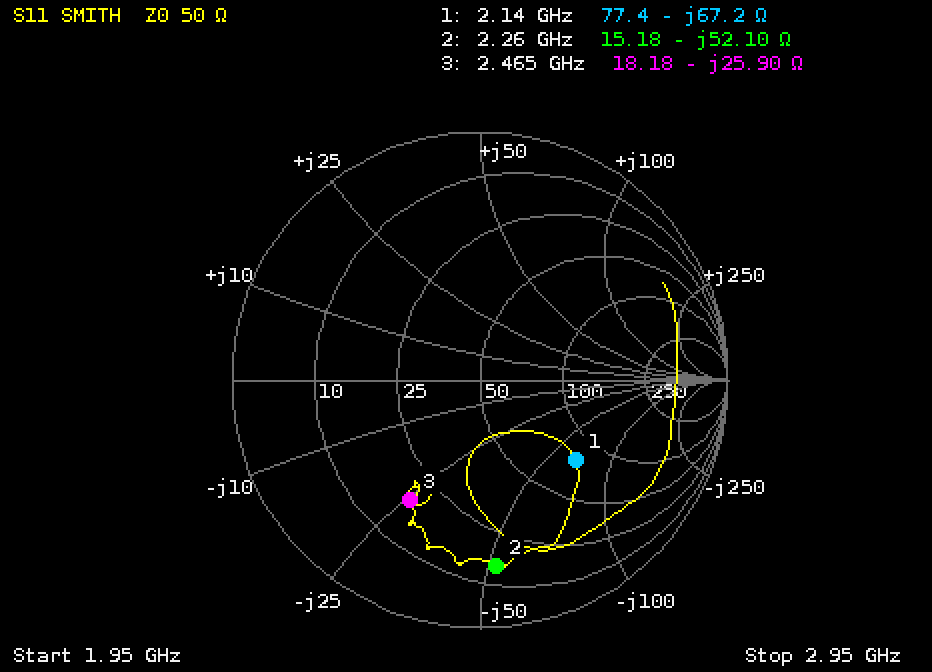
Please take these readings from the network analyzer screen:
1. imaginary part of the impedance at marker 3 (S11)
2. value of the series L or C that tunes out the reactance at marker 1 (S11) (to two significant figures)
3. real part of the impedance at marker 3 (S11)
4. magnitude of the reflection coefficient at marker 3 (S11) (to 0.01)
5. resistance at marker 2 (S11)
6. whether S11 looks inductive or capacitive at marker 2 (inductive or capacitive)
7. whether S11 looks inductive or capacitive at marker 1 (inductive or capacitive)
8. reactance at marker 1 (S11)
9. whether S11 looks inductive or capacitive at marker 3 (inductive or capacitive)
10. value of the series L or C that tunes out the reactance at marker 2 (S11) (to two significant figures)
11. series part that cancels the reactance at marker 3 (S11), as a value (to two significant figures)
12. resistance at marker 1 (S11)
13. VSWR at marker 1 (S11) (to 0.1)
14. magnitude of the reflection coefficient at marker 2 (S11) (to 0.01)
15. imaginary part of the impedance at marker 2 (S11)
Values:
-25.90 Ω
5.0 nH
18.18 Ω
0.56
15.18 Ω
capacitive
capacitive
-67.2 Ω
capacitive
3.7 nH
1.7 nH
77.4 Ω
3.0
0.75
-52.10 Ω
